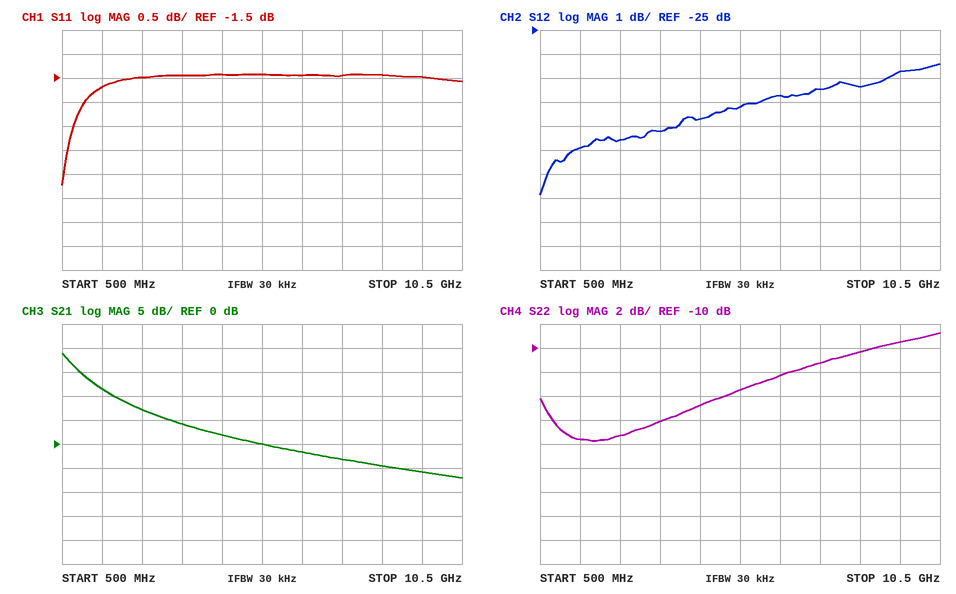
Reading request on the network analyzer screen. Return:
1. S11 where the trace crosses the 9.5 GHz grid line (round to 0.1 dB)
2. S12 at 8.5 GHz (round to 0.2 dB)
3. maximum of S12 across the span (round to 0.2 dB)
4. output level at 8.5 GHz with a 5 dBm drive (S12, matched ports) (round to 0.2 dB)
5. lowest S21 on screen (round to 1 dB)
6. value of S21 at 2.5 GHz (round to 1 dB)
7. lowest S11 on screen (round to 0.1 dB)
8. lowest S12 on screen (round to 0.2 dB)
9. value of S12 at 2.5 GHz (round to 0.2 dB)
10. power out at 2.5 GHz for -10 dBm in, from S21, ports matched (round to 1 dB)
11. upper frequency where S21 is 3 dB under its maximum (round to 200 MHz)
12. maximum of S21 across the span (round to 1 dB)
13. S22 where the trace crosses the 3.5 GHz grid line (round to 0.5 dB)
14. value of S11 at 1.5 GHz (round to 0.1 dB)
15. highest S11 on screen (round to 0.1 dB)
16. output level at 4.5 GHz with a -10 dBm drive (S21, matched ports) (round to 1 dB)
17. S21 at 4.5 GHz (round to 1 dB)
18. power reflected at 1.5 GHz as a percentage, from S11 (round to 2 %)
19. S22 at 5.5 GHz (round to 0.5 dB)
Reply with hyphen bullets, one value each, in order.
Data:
- -1.5 dB
- -27.4 dB
- -26.4 dB
- -22.4 dBm
- -7 dB
- 7 dB
- -3.7 dB
- -31.8 dB
- -29.6 dB
- -3 dBm
- 800 MHz
- 19 dB
- -16.0 dB
- -1.7 dB
- -1.4 dB
- -8 dBm
- 2 dB
- 68 %
- -13.5 dB
